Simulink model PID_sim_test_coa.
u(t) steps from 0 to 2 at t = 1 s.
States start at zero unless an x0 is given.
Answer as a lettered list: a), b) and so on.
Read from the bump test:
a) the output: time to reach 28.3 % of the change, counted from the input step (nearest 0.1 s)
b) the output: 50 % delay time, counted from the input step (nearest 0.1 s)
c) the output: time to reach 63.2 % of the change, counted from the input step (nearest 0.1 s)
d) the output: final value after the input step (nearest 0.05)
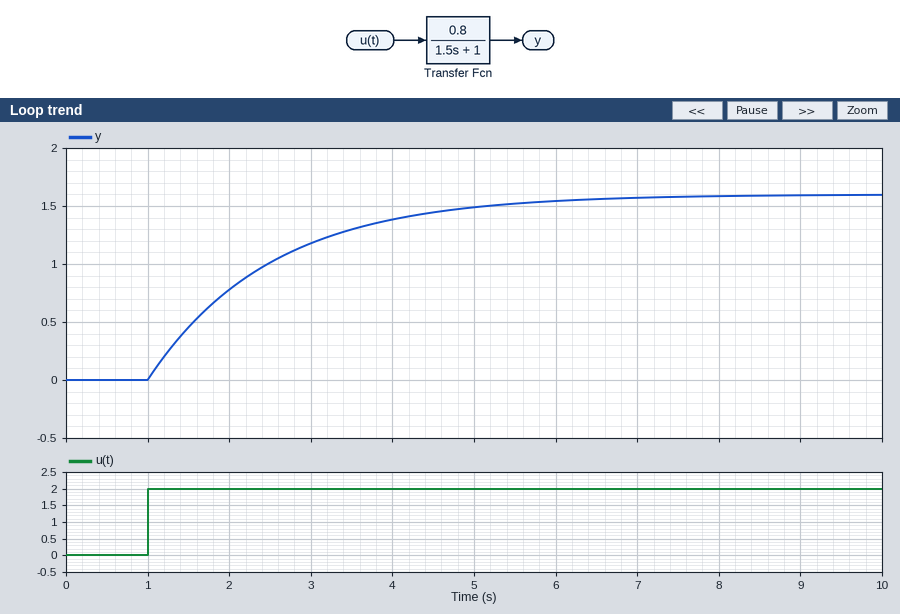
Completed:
a) 0.5 s
b) 1.0 s
c) 1.5 s
d) 1.60
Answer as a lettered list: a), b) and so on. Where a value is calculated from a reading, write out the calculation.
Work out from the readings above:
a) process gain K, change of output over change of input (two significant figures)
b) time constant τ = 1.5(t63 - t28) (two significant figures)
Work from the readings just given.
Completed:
a) (1.6 - 0) / 2 = 0.80
b) 1.5 × (1.5 - 0.5) = 1.5 s
